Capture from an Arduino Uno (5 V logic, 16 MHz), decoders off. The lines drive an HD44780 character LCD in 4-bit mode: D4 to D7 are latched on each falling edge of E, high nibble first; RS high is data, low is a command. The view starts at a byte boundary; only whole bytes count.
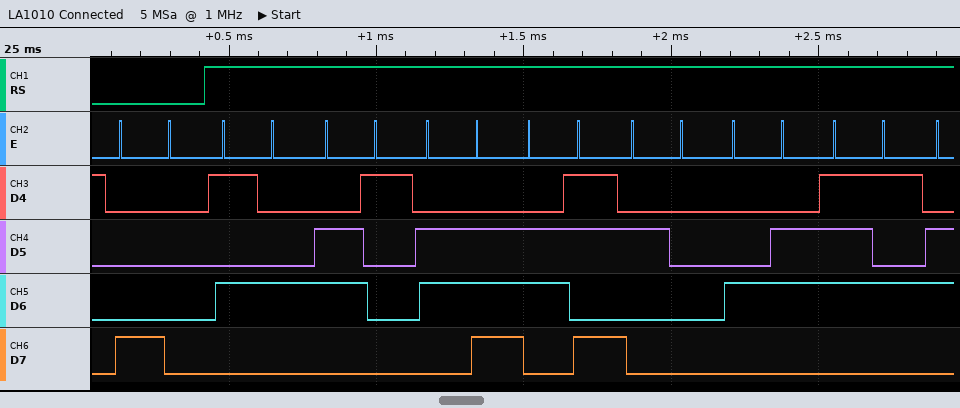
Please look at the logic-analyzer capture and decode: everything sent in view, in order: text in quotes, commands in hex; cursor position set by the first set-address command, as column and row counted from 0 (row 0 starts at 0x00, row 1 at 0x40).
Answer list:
0x80 "Tank Fu"
column 0, row 0
